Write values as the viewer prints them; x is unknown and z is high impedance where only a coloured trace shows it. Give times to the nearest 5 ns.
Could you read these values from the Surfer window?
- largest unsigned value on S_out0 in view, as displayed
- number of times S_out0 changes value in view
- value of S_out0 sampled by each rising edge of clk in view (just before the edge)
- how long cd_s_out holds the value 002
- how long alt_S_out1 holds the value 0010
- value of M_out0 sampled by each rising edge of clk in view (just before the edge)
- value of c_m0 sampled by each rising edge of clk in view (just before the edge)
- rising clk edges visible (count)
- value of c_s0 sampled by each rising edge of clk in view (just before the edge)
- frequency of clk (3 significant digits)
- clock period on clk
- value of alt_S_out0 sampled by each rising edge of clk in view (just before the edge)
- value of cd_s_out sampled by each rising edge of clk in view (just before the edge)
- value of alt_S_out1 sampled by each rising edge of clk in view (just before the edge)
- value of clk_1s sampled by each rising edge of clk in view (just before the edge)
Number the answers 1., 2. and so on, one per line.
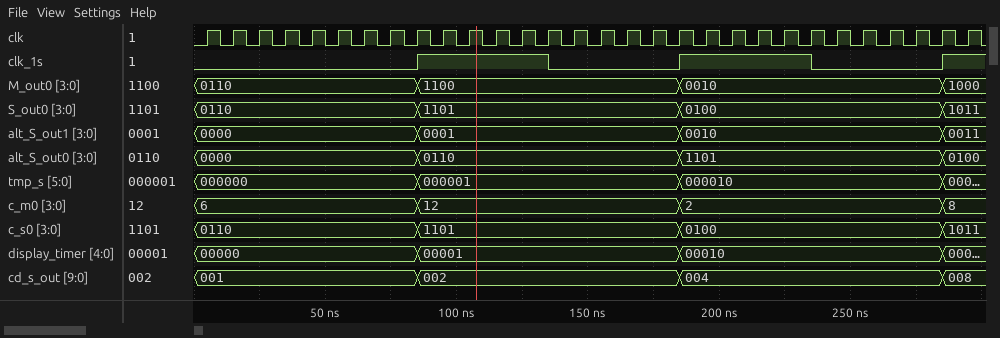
1. 1101
2. 3
3. 0110, 0110, 0110, 0110, 0110, 0110, 0110, 0110, 0110, 1101, 1101, 1101, 1101, 1101, 1101, 1101, 1101, 1101, 1101, 0100, 0100, 0100, 0100, 0100, 0100, 0100, 0100, 0100, 0100, 1011
4. 100 ns
5. 100 ns
6. 0110, 0110, 0110, 0110, 0110, 0110, 0110, 0110, 0110, 1100, 1100, 1100, 1100, 1100, 1100, 1100, 1100, 1100, 1100, 0010, 0010, 0010, 0010, 0010, 0010, 0010, 0010, 0010, 0010, 1000
7. 6, 6, 6, 6, 6, 6, 6, 6, 6, 12, 12, 12, 12, 12, 12, 12, 12, 12, 12, 2, 2, 2, 2, 2, 2, 2, 2, 2, 2, 8
8. 30
9. 0110, 0110, 0110, 0110, 0110, 0110, 0110, 0110, 0110, 1101, 1101, 1101, 1101, 1101, 1101, 1101, 1101, 1101, 1101, 0100, 0100, 0100, 0100, 0100, 0100, 0100, 0100, 0100, 0100, 1011
10. 100 MHz
11. 10 ns
12. 0000, 0000, 0000, 0000, 0000, 0000, 0000, 0000, 0000, 0110, 0110, 0110, 0110, 0110, 0110, 0110, 0110, 0110, 0110, 1101, 1101, 1101, 1101, 1101, 1101, 1101, 1101, 1101, 1101, 0100
13. 001, 001, 001, 001, 001, 001, 001, 001, 001, 002, 002, 002, 002, 002, 002, 002, 002, 002, 002, 004, 004, 004, 004, 004, 004, 004, 004, 004, 004, 008
14. 0000, 0000, 0000, 0000, 0000, 0000, 0000, 0000, 0000, 0001, 0001, 0001, 0001, 0001, 0001, 0001, 0001, 0001, 0001, 0010, 0010, 0010, 0010, 0010, 0010, 0010, 0010, 0010, 0010, 0011
15. 0 0 0 0 0 0 0 0 0 1 1 1 1 1 0 0 0 0 0 1 1 1 1 1 0 0 0 0 0 1
